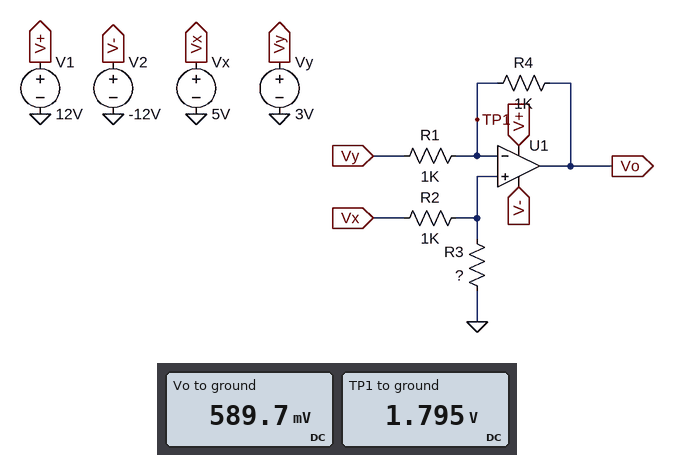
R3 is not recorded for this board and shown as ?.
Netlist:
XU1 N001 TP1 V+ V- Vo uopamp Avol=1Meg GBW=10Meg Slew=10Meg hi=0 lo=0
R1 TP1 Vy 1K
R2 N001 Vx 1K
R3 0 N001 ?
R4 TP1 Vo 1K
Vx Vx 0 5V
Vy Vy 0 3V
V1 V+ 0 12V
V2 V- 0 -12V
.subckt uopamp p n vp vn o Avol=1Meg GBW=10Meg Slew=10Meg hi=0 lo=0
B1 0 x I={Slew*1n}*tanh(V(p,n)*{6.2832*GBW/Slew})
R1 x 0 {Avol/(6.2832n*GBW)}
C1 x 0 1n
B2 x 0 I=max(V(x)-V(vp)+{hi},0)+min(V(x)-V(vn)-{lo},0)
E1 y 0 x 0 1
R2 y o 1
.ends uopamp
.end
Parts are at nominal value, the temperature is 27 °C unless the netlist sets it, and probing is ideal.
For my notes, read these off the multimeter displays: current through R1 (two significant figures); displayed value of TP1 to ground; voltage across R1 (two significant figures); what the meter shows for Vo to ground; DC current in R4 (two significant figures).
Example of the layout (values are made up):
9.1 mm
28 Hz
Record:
1.2 mA
1.795 V
1.2 V
589.7 mV
1.2 mA
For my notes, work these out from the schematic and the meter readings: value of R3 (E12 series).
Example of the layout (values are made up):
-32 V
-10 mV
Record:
560 Ω
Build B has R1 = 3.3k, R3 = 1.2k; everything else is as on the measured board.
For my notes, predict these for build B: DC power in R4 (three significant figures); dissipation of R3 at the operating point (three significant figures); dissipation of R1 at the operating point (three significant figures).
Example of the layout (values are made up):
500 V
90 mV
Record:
6.83 µW
6.20 mW
22.5 µW
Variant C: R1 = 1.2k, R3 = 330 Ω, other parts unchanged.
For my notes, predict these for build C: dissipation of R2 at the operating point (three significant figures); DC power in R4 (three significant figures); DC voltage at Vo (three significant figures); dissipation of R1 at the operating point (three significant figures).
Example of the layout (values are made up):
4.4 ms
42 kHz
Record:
14.1 mW
2.15 mW
-226 mV
2.58 mW
